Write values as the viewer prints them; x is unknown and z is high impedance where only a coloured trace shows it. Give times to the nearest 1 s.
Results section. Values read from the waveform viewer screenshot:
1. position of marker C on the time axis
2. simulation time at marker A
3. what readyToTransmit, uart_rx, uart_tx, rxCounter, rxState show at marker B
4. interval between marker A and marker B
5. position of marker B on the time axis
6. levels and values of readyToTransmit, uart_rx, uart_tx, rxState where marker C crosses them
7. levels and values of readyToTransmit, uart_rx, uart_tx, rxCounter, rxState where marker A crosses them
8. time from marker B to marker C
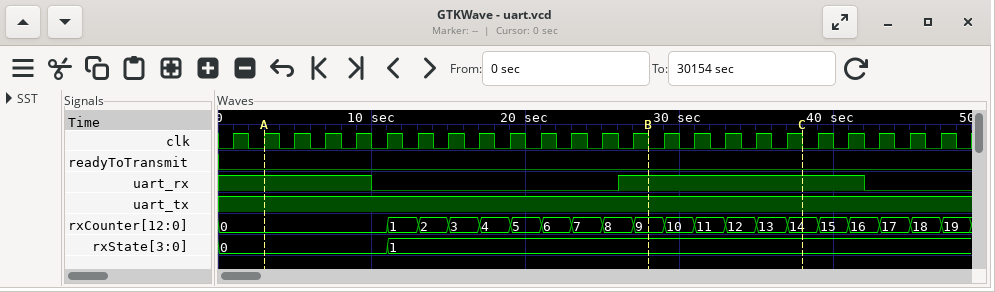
38 s
3 s
readyToTransmit=0, uart_rx=1, uart_tx=1, rxCounter=9, rxState=1
25 s
28 s
readyToTransmit=0, uart_rx=1, uart_tx=1, rxState=1
readyToTransmit=0, uart_rx=1, uart_tx=1, rxCounter=0, rxState=0
10 s
